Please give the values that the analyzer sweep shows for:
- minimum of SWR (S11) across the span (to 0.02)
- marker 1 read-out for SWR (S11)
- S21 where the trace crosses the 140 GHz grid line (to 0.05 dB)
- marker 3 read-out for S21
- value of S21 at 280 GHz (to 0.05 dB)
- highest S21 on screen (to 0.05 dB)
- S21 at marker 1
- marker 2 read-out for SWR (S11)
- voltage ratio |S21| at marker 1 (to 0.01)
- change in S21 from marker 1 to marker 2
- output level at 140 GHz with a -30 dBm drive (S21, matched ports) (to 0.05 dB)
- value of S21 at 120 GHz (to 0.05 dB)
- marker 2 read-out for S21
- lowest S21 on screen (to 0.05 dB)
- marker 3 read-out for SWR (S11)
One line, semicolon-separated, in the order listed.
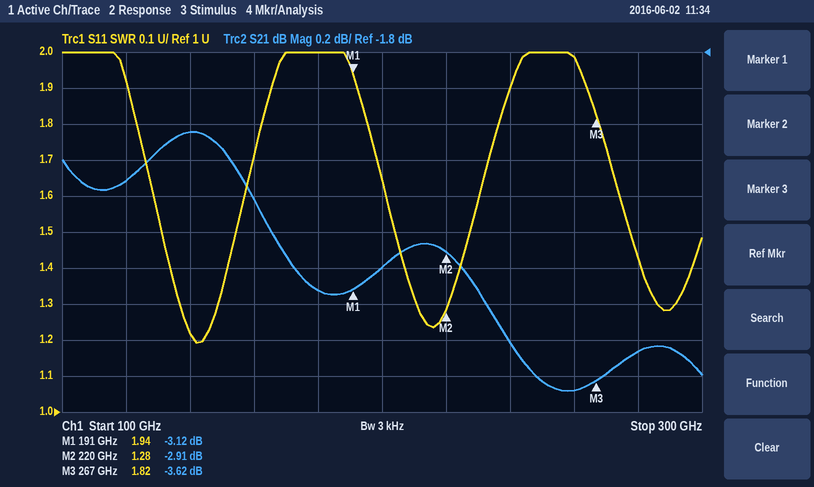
1.20; 1.94; -2.25 dB; -3.62 dB; -3.45 dB; -2.25 dB; -3.12 dB; 1.28; 0.70; 0.21 dB; -32.25 dBm; -2.50 dB; -2.91 dB; -3.70 dB; 1.82
